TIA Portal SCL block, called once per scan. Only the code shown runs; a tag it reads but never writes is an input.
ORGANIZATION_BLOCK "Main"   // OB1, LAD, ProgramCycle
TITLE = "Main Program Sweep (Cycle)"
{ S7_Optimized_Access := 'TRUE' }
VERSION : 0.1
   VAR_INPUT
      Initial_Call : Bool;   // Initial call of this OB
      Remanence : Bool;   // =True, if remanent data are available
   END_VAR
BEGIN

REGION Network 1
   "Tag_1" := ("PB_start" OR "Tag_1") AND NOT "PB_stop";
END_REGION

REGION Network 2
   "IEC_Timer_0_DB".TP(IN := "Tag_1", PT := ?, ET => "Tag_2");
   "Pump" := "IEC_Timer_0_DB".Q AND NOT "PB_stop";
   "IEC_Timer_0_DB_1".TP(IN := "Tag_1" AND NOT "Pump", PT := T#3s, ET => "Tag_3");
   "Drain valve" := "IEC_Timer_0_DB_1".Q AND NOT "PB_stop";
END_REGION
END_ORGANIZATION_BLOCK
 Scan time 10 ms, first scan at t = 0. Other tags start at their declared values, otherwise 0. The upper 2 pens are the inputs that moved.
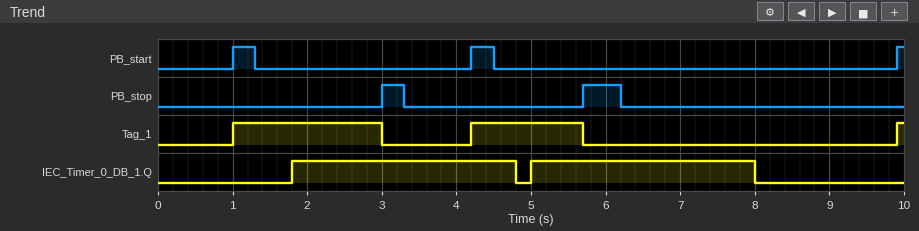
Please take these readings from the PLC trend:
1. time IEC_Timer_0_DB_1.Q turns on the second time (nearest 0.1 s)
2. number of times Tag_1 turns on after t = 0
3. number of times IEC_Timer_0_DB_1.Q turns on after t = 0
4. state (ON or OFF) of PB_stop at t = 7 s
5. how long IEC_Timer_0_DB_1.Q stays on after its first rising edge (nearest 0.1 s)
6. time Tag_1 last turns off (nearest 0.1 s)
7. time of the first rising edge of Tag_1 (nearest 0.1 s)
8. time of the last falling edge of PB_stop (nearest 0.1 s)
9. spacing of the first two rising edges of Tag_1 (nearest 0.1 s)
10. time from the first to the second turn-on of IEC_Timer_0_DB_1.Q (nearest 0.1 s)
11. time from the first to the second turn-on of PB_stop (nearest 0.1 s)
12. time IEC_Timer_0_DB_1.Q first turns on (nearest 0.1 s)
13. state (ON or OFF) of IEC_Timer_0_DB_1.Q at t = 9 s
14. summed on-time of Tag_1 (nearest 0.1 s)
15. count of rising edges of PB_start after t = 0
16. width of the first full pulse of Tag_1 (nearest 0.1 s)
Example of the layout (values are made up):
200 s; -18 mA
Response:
5.0 s; 3; 2; OFF; 3.0 s; 5.7 s; 1.0 s; 6.2 s; 3.2 s; 3.2 s; 2.7 s; 1.8 s; OFF; 3.6 s; 3; 2.0 s
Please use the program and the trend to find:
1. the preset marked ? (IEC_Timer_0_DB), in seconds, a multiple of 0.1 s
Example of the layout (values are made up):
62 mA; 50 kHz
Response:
0.8 s
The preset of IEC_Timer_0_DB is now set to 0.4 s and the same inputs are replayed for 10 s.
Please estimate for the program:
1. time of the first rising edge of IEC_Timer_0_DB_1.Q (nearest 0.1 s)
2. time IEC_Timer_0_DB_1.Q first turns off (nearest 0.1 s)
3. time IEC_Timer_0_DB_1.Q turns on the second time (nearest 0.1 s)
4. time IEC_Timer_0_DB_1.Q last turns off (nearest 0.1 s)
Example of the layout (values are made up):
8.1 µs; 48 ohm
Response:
1.4 s; 4.4 s; 4.6 s; 7.6 s
